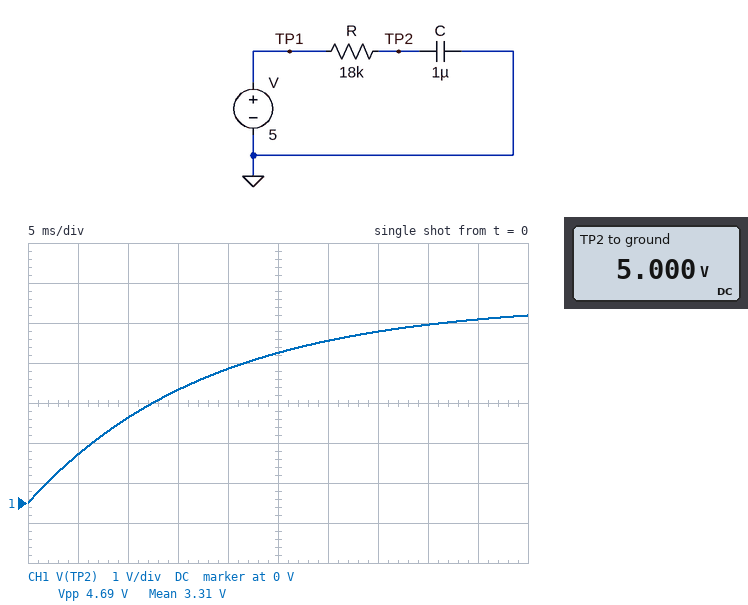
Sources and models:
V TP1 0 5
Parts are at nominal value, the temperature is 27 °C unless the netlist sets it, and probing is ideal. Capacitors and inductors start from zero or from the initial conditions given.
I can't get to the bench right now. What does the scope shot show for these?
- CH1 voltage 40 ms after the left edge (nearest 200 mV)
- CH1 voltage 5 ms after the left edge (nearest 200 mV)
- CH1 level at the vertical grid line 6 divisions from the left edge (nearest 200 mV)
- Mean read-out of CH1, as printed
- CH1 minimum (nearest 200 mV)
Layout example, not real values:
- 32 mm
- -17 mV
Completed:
- 4.4 V
- 1.2 V
- 4.0 V
- 3.31 V
- 0 V
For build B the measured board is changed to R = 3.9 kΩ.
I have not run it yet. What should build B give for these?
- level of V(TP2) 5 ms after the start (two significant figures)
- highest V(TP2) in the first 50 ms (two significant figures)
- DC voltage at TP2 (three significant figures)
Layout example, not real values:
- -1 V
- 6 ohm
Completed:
- 3.6 V
- 5.0 V
- 5.00 V
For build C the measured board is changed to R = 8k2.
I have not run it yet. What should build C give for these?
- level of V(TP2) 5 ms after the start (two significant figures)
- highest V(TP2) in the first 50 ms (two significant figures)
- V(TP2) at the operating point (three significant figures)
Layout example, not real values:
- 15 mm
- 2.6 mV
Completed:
- 2.3 V
- 5.0 V
- 5.00 V
